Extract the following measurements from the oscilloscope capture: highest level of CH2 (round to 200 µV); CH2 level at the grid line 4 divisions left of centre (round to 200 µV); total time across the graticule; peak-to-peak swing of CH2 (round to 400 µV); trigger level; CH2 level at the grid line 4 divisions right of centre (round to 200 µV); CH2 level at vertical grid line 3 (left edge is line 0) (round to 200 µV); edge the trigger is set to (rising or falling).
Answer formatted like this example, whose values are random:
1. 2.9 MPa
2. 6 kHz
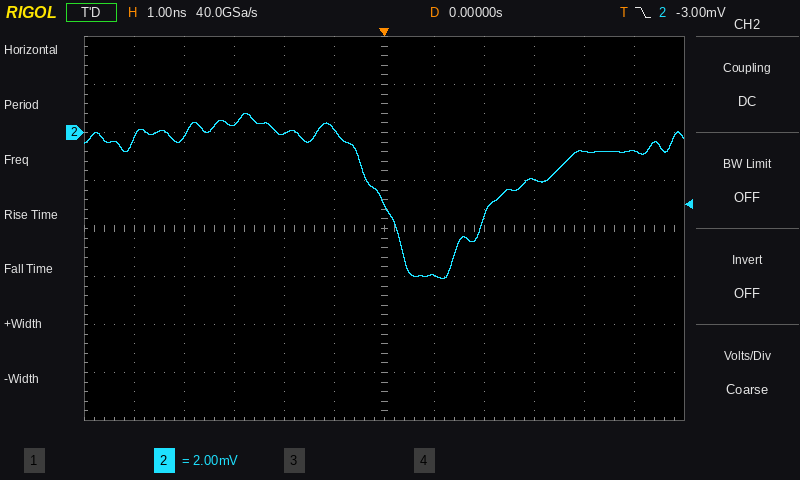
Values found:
1. 800 µV
2. -200 µV
3. 12 ns
4. 6.8 mV
5. -3.00 mV
6. -800 µV
7. 400 µV
8. falling
